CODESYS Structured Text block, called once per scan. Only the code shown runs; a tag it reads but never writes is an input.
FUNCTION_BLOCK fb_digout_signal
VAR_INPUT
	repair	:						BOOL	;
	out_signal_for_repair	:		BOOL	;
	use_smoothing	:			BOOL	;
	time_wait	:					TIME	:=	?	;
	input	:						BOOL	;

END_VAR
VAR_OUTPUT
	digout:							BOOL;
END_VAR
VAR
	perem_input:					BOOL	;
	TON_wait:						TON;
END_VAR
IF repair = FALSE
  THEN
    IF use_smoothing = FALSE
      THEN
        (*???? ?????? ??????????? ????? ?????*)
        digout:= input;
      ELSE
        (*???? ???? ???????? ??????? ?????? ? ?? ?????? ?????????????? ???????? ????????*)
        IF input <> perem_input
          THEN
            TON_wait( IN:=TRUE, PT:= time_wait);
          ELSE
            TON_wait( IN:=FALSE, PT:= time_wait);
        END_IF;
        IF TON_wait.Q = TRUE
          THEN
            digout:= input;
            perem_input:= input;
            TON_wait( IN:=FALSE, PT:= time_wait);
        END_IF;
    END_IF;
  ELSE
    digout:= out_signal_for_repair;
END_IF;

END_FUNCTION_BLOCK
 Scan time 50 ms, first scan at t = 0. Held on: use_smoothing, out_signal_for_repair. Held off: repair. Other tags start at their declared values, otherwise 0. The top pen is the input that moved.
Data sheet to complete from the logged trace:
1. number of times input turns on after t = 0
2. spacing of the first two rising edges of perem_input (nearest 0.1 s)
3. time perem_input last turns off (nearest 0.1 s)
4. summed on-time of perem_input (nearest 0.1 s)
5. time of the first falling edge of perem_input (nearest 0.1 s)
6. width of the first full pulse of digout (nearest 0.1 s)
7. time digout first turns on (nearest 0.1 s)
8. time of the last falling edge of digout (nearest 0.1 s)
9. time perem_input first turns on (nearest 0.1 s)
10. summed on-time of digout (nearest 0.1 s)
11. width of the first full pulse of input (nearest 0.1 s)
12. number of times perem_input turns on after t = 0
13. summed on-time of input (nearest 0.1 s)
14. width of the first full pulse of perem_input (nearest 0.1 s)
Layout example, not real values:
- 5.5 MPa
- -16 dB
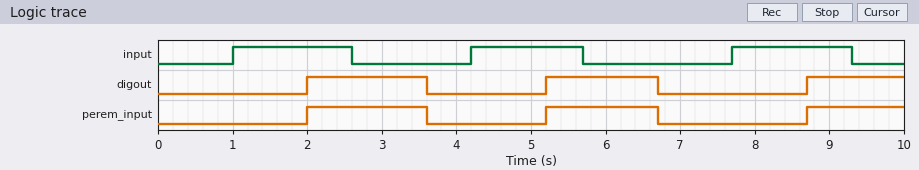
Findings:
- 3
- 3.2 s
- 6.7 s
- 4.4 s
- 3.6 s
- 1.6 s
- 2.0 s
- 6.7 s
- 2.0 s
- 4.4 s
- 1.6 s
- 3
- 4.7 s
- 1.6 s
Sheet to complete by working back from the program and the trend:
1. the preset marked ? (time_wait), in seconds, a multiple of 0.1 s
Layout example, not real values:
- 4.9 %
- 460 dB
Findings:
- 1.0 s
